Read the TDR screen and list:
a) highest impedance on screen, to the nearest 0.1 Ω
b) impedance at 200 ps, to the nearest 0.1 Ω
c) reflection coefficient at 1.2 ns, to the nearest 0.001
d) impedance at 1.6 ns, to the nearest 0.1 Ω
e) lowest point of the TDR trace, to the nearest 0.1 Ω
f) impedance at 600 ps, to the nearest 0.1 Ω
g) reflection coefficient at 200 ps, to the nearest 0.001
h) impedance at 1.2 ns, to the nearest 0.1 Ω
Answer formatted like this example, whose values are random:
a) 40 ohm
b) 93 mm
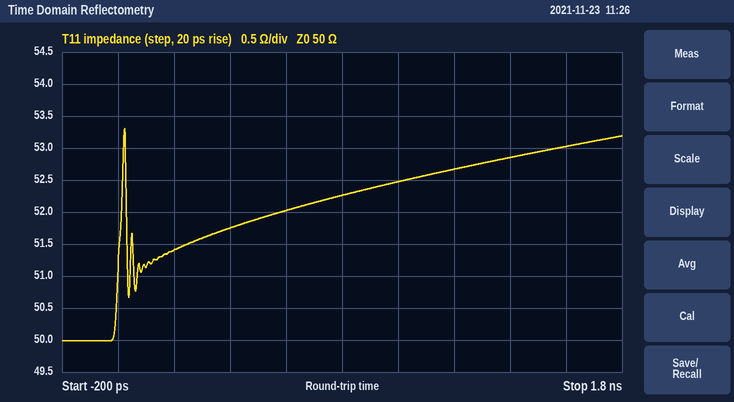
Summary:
a) 53.3 Ω
b) 51.4 Ω
c) +0.026
d) 53.0 Ω
e) 50.0 Ω
f) 52.0 Ω
g) +0.014
h) 52.7 Ω
